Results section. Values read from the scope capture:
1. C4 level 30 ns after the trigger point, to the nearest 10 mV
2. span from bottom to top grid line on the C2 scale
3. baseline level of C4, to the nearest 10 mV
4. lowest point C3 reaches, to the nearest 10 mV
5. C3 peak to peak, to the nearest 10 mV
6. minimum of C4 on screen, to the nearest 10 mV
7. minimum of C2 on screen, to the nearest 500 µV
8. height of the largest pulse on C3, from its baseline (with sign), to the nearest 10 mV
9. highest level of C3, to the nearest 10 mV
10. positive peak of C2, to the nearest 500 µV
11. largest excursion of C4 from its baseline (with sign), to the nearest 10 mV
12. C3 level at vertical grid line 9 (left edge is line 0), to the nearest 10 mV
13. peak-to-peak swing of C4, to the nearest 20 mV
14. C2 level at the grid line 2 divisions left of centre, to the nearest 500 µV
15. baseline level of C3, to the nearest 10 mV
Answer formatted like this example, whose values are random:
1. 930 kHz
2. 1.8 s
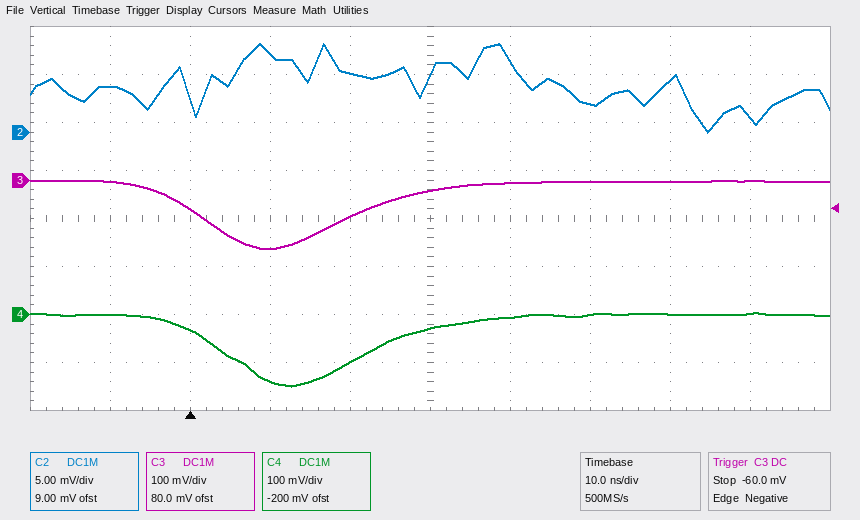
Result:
1. -30 mV
2. 40 mV
3. 0 mV
4. -140 mV
5. 140 mV
6. -150 mV
7. 0.0 mV
8. -140 mV
9. 0 mV
10. 9.0 mV
11. -150 mV
12. 0 mV
13. 160 mV
14. 8.0 mV
15. 0 mV
